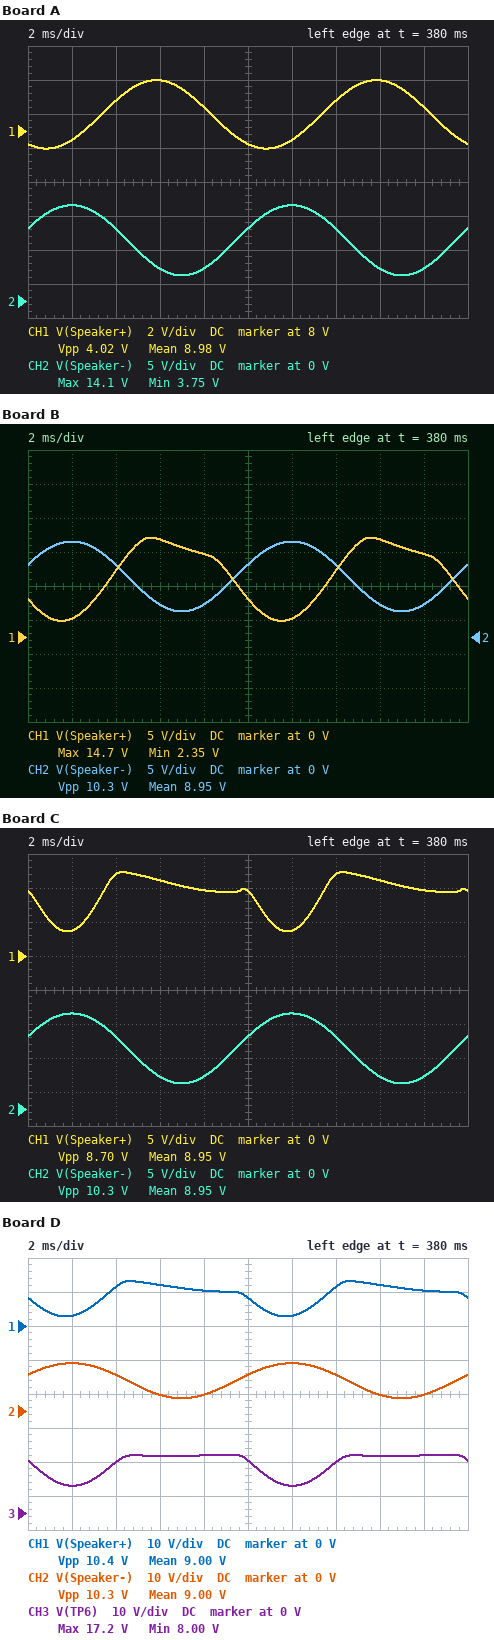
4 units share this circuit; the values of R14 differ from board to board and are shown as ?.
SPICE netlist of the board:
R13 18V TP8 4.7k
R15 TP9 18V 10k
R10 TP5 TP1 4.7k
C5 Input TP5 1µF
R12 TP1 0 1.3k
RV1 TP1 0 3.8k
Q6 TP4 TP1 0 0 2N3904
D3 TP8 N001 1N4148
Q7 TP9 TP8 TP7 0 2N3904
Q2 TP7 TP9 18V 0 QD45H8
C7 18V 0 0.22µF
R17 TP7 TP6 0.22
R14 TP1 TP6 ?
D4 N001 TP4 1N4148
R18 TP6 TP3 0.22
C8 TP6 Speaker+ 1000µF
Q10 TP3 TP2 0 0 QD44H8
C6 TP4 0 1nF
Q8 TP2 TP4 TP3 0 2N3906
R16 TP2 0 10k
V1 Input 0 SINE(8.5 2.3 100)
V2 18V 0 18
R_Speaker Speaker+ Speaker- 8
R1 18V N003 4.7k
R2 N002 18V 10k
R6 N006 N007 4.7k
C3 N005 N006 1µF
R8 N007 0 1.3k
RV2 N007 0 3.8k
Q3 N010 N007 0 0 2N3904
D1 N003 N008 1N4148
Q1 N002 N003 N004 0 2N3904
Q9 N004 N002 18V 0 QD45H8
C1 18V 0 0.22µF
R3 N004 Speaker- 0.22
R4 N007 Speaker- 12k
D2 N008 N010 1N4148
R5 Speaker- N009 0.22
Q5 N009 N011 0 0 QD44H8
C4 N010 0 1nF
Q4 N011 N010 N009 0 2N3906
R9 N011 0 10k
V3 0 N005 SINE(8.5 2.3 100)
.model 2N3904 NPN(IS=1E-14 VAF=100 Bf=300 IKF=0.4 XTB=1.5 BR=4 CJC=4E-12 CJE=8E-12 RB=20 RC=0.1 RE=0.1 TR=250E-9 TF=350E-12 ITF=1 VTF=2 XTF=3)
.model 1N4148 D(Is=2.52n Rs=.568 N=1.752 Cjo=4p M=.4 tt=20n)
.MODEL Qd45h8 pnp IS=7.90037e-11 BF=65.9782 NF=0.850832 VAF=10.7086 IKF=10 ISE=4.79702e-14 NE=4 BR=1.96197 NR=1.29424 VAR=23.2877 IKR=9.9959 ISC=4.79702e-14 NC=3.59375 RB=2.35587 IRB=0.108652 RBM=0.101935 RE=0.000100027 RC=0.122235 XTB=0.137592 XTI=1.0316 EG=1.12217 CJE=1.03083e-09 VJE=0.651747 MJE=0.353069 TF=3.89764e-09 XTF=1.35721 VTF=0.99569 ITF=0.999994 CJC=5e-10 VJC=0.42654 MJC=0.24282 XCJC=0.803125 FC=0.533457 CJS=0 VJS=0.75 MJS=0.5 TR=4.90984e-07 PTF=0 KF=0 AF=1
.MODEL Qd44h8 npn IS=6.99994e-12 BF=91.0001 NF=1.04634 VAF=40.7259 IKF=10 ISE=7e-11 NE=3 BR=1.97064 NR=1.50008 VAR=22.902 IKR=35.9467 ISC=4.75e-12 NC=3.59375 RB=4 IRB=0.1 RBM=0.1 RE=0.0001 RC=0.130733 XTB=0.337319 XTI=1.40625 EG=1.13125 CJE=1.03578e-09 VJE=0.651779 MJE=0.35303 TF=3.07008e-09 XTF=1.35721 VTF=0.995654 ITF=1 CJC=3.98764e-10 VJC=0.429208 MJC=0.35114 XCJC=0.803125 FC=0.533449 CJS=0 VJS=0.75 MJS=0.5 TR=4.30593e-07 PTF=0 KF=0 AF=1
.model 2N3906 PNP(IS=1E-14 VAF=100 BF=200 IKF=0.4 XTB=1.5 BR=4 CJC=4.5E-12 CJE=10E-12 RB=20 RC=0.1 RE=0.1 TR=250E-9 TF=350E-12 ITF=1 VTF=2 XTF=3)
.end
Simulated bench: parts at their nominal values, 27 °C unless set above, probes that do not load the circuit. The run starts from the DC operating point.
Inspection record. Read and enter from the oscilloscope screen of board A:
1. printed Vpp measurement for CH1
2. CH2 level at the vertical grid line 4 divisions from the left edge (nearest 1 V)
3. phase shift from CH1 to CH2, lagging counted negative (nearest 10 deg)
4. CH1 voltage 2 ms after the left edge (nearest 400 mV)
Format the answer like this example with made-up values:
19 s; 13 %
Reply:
4.02 V; 5 V; 140 deg; 7.6 V
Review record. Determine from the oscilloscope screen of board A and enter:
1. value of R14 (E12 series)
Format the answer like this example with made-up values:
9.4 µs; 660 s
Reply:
3.9 kΩ
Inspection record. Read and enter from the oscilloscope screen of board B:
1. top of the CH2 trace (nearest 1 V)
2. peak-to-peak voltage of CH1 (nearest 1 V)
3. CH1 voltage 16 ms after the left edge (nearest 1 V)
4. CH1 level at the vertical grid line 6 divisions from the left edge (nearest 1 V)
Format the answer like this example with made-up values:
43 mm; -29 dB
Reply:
14 V; 12 V; 14 V; 3 V
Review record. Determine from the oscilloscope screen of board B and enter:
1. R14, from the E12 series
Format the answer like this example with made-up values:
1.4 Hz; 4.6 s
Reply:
18 kΩ
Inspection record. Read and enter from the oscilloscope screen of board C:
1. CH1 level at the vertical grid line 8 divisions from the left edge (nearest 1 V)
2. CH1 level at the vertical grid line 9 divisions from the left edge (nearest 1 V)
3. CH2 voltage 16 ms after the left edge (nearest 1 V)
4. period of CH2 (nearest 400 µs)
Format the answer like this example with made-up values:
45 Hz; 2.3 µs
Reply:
11 V; 10 V; 5 V; 10.0 ms
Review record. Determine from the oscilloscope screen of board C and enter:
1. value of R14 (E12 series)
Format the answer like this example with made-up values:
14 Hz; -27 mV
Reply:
33 kΩ
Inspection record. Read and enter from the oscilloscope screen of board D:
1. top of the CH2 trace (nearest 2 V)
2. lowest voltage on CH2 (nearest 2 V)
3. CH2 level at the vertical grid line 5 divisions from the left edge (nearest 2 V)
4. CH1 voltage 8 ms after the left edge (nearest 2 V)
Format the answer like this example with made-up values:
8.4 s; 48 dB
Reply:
14 V; 4 V; 10 V; 10 V
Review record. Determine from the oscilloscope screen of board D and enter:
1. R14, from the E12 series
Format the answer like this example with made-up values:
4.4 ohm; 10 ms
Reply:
27 kΩ
